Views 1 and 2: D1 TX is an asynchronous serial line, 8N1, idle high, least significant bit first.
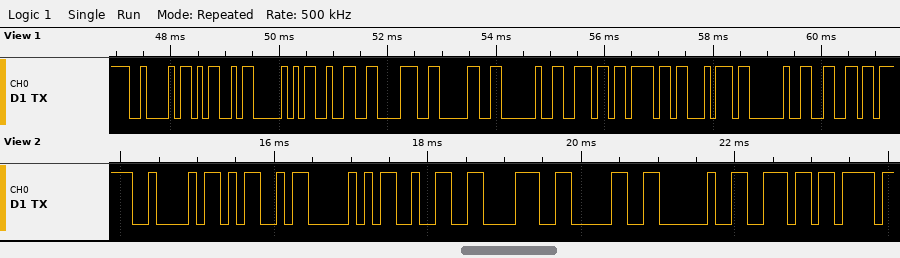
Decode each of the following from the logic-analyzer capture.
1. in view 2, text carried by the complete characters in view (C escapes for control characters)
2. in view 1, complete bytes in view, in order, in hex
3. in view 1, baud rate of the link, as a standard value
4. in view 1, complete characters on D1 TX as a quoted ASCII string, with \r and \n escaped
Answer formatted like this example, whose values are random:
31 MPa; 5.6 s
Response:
"BMP280 n"; 42 4D 50 32 38 30 20 6E 6F 74 20 66; 9600 baud; "BMP280 not f"
